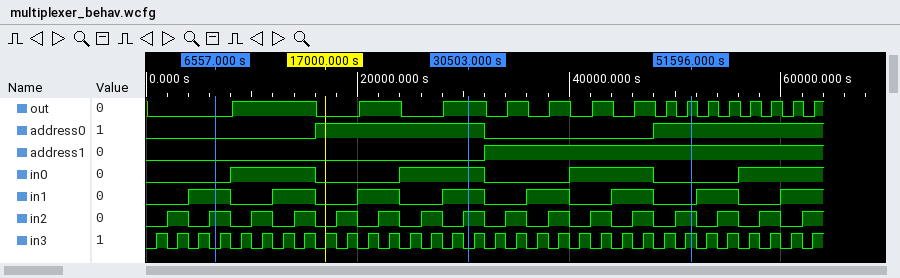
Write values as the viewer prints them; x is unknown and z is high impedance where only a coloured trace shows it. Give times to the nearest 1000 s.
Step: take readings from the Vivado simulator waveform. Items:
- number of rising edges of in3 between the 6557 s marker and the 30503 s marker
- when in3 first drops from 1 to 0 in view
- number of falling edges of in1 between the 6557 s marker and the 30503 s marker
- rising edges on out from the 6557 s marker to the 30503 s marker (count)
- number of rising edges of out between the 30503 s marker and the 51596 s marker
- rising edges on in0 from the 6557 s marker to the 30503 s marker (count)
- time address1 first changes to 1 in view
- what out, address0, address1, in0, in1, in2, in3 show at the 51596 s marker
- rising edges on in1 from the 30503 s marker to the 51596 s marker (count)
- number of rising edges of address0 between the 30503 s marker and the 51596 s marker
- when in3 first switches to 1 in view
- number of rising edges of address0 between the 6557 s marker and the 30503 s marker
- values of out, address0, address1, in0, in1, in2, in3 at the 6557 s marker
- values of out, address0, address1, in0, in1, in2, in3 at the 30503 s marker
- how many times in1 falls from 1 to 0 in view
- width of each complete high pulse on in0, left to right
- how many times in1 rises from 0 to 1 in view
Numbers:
12
2000 s
3
3
6
2
32000 s
out=1, address0=1, address1=1, in0=0, in1=0, in2=1, in3=1
2
1
1000 s
1
out=0, address0=0, address1=0, in0=0, in1=1, in2=1, in3=0
out=1, address0=1, address1=0, in0=1, in1=1, in2=1, in3=0
7
8000 s, 8000 s, 8000 s
8
